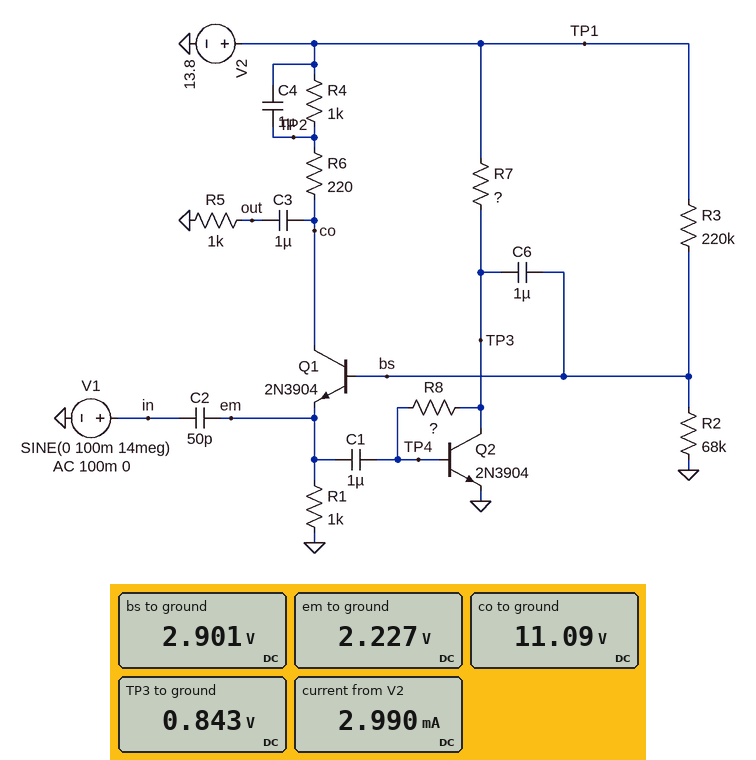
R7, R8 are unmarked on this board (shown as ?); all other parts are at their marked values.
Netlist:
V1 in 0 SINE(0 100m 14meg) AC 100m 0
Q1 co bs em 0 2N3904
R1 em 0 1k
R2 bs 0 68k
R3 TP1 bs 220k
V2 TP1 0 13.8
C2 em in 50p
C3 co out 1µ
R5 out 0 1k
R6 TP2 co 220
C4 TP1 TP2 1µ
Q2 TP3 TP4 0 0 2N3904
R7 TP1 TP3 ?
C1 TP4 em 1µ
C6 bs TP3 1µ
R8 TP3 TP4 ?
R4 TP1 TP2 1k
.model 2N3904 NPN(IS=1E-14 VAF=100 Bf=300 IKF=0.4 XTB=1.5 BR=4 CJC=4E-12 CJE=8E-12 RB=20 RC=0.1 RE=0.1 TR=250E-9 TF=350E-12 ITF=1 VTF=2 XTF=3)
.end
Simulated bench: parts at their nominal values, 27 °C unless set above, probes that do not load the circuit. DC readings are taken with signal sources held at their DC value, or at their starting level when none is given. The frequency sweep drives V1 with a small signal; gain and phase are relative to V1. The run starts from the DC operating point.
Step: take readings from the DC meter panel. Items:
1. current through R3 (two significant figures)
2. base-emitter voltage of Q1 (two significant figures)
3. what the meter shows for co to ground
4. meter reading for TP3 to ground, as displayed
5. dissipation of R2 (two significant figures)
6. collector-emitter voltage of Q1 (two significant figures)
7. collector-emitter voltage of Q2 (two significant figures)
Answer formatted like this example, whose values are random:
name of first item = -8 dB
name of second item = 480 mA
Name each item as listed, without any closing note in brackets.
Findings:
current through R3 = 50 µA
base-emitter voltage of Q1 = 670 mV
what the meter shows for co to ground = 11.09 V
meter reading for TP3 to ground, as displayed = 0.843 V
dissipation of R2 = 120 µW
collector-emitter voltage of Q1 = 8.9 V
collector-emitter voltage of Q2 = 840 mV
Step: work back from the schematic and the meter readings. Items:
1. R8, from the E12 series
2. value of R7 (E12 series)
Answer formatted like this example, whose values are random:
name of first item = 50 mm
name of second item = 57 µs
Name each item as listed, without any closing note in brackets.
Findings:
R8, from the E12 series = 82 kΩ
value of R7 = 18 kΩ
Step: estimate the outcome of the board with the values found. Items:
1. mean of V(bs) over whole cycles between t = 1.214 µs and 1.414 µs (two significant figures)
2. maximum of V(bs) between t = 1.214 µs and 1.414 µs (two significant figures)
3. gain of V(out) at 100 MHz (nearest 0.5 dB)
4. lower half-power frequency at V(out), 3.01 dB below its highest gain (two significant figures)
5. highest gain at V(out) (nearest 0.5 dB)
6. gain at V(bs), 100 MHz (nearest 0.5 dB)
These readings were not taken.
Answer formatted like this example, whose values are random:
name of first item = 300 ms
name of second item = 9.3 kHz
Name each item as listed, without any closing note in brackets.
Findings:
mean of V(bs) over whole cycles between t = 1.214 µs and 1.414 µs = 2.9 V
maximum of V(bs) between t = 1.214 µs and 1.414 µs = 2.9 V
gain of V(out) at 100 MHz = 26.0 dB
lower half-power frequency at V(out), 3.01 dB below its highest gain = 89 MHz
highest gain at V(out) = 26.0 dB
gain at V(bs), 100 MHz = 7.5 dB
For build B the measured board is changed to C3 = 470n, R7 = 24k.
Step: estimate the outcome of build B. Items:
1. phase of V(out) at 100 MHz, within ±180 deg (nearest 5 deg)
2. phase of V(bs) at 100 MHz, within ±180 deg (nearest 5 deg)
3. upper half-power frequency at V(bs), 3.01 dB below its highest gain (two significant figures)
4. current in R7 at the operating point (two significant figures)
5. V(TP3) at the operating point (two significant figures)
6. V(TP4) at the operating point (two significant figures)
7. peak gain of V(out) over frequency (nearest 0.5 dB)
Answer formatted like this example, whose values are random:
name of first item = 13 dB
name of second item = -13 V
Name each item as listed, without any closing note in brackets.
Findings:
phase of V(out) at 100 MHz, within ±180 deg = -55 deg
phase of V(bs) at 100 MHz, within ±180 deg = 90 deg
upper half-power frequency at V(bs), 3.01 dB below its highest gain = 110 MHz
current in R7 at the operating point = 540 µA
V(TP3) at the operating point = 790 mV
V(TP4) at the operating point = 640 mV
peak gain of V(out) over frequency = 25.0 dB
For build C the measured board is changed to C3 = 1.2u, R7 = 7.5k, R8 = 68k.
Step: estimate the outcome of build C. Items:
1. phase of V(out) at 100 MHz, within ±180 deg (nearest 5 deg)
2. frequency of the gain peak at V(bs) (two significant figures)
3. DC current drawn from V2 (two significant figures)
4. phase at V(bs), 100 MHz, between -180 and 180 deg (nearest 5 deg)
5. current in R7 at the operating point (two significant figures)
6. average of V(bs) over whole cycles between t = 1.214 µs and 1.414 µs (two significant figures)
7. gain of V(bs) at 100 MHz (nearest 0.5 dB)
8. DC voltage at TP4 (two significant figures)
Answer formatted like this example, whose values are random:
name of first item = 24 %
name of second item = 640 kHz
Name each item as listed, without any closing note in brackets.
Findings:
phase of V(out) at 100 MHz, within ±180 deg = 50 deg
frequency of the gain peak at V(bs) = 140 MHz
DC current drawn from V2 = 4.0 mA
phase at V(bs), 100 MHz, between -180 and 180 deg = -115 deg
current in R7 at the operating point = 1.7 mA
average of V(bs) over whole cycles between t = 1.214 µs and 1.414 µs = 2.9 V
gain of V(bs) at 100 MHz = -0.5 dB
DC voltage at TP4 = 670 mV
